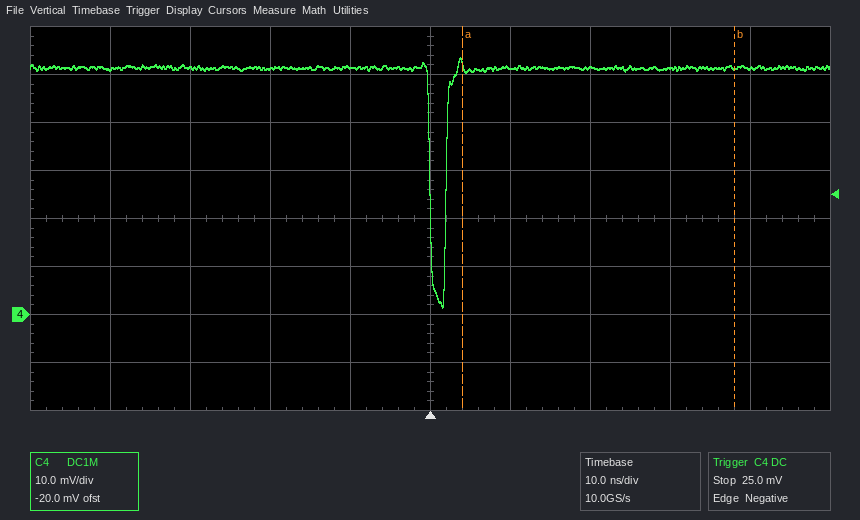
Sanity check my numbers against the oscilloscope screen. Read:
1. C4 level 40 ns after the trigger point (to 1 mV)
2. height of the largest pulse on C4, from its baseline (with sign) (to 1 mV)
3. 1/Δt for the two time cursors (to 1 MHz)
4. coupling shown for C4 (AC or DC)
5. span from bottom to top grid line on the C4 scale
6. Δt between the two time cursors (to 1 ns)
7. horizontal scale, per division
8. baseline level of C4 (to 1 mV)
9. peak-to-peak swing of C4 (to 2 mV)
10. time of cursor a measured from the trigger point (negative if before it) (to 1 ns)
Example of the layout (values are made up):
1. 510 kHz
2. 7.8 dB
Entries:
1. 51 mV
2. -50 mV
3. 29 MHz
4. DC
5. 80 mV
6. 34 ns
7. 10 ns
8. 51 mV
9. 52 mV
10. +4 ns
